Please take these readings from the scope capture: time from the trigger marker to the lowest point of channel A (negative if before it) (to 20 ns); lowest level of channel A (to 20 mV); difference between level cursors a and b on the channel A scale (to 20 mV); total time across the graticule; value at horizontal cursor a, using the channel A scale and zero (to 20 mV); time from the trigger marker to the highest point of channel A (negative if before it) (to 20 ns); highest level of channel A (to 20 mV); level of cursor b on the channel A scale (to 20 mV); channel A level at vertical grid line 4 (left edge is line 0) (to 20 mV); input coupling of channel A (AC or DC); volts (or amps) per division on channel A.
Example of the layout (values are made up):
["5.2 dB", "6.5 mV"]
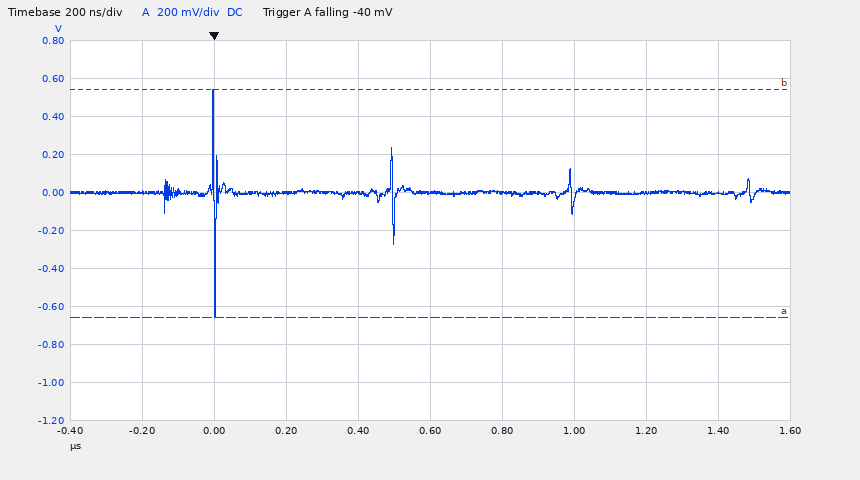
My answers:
["0 ns", "-660 mV", "1.20 V", "2 µs", "-660 mV", "0 ns", "540 mV", "540 mV", "0 mV", "DC", "200 mV"]
